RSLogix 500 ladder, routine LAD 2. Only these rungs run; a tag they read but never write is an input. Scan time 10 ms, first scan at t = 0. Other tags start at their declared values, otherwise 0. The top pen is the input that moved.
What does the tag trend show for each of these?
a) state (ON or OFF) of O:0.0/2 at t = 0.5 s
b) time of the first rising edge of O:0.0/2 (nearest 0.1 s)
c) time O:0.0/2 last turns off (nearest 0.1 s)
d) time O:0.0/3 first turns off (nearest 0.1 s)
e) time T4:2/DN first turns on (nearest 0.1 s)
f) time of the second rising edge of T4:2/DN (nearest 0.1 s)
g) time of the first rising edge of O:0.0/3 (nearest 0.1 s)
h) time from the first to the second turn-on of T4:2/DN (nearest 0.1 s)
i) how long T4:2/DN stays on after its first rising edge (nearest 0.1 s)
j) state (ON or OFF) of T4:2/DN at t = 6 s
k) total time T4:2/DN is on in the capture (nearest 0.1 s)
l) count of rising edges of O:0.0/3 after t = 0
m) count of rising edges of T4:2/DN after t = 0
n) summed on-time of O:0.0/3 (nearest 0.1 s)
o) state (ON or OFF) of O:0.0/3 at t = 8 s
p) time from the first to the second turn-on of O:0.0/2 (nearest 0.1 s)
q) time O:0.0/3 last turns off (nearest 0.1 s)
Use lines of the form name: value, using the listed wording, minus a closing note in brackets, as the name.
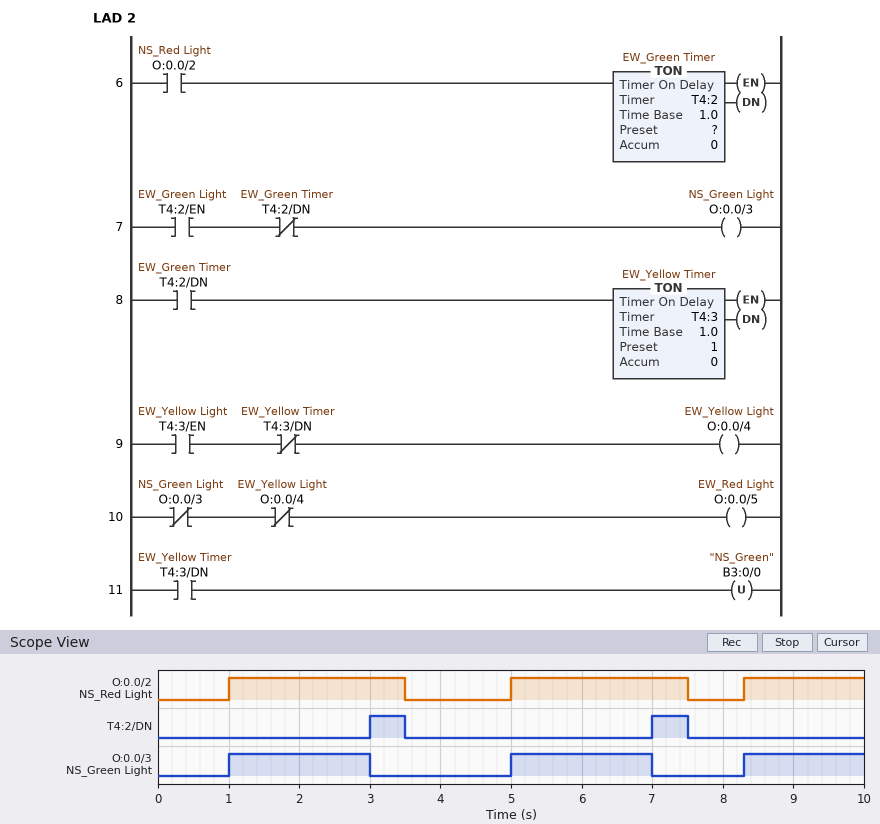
state (ON or OFF) of O:0.0/2 at t = 0.5 s: OFF
time of the first rising edge of O:0.0/2: 1.0 s
time O:0.0/2 last turns off: 7.5 s
time O:0.0/3 first turns off: 3.0 s
time T4:2/DN first turns on: 3.0 s
time of the second rising edge of T4:2/DN: 7.0 s
time of the first rising edge of O:0.0/3: 1.0 s
time from the first to the second turn-on of T4:2/DN: 4.0 s
how long T4:2/DN stays on after its first rising edge: 0.5 s
state (ON or OFF) of T4:2/DN at t = 6 s: OFF
total time T4:2/DN is on in the capture: 1.0 s
count of rising edges of O:0.0/3 after t = 0: 3
count of rising edges of T4:2/DN after t = 0: 2
summed on-time of O:0.0/3: 5.7 s
state (ON or OFF) of O:0.0/3 at t = 8 s: OFF
time from the first to the second turn-on of O:0.0/2: 4.0 s
time O:0.0/3 last turns off: 7.0 s
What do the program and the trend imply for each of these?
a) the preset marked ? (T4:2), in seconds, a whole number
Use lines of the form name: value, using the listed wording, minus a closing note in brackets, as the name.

the preset marked ? (T4:2), in seconds, a whole number: 2 s
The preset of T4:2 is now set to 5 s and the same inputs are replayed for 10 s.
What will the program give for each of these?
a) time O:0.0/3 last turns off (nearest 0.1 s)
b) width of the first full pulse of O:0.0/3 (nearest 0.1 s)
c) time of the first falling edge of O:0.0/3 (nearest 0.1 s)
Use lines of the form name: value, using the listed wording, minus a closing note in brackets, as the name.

time O:0.0/3 last turns off: 7.5 s
width of the first full pulse of O:0.0/3: 2.5 s
time of the first falling edge of O:0.0/3: 3.5 s
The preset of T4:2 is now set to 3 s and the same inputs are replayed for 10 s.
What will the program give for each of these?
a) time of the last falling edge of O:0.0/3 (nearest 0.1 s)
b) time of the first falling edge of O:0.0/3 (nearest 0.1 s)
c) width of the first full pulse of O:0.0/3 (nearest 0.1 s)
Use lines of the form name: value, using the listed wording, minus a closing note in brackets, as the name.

time of the last falling edge of O:0.0/3: 7.5 s
time of the first falling edge of O:0.0/3: 3.5 s
width of the first full pulse of O:0.0/3: 2.5 s
